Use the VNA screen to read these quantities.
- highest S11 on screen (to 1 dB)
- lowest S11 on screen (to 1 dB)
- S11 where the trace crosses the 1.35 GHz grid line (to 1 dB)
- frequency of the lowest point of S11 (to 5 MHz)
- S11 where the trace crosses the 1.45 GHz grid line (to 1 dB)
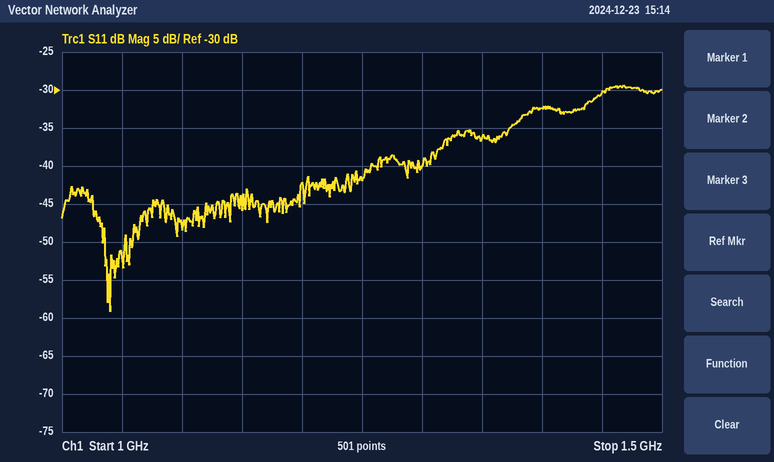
-29 dB
-59 dB
-36 dB
1.040 GHz
-30 dB
